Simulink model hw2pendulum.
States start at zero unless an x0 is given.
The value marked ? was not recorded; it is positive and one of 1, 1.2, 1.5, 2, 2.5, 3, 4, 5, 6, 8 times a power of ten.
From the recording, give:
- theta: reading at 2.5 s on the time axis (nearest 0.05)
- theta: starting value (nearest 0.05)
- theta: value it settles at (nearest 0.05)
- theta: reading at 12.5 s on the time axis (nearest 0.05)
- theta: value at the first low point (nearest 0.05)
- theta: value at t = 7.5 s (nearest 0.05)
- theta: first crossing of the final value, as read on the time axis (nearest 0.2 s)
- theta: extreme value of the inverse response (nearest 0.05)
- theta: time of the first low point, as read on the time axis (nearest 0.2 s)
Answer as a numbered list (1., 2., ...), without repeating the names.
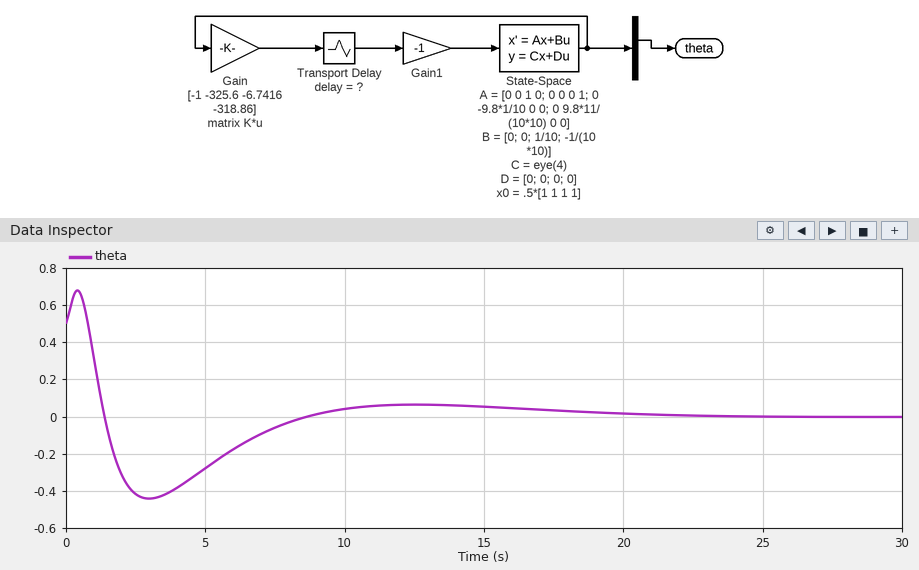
1. -0.40
2. 0.50
3. 0.00
4. 0.05
5. -0.45
6. -0.05
7. 1.4 s
8. 0.70
9. 3.0 s
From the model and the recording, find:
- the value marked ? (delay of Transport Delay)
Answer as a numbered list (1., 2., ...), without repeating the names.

1. 0.2
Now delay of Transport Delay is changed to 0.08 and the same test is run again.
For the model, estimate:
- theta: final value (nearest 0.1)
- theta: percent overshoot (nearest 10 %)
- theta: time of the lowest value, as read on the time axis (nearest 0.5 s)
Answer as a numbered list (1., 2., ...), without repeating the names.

1. 0.0
2. 80 %
3. 3.5 s
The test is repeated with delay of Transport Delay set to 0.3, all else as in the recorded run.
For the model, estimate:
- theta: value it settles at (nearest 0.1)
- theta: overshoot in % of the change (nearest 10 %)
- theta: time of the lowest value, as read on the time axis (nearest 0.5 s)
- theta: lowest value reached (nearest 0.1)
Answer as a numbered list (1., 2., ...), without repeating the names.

1. 0.0
2. 100 %
3. 2.0 s
4. -0.5
